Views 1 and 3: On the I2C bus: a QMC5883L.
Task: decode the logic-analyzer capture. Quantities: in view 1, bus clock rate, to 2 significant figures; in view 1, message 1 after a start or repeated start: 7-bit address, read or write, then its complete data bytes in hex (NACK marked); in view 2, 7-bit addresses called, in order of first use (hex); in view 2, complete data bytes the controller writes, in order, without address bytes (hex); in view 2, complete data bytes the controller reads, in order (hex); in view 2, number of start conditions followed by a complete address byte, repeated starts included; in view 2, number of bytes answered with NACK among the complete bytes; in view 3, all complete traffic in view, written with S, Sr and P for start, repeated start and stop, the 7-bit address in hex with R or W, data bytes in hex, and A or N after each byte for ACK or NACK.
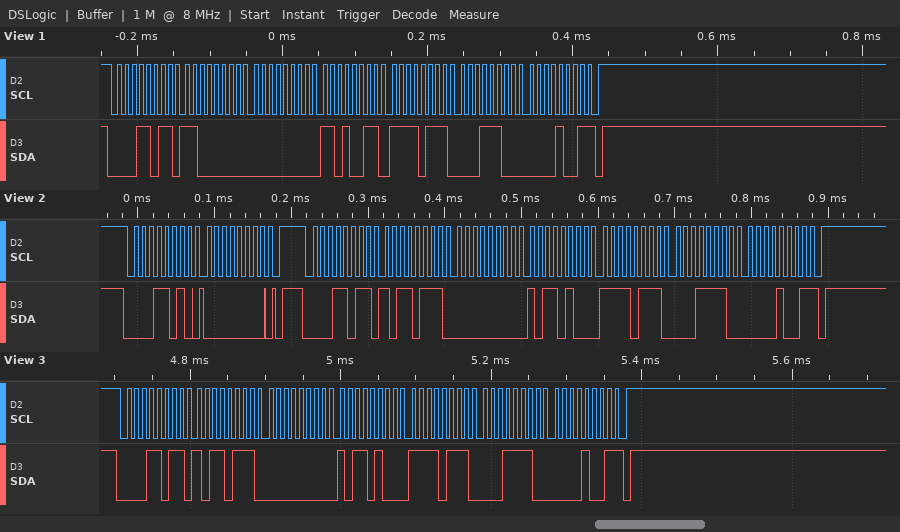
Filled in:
100 kHz
0x0D read: C0 00 D3 F7 1C 09 NACK
0x0D
00
B7 00 B4 F7 1E 09
2
1
S 0DR A B7 A 00 A B4 A F7 A 1E A 09 N P
